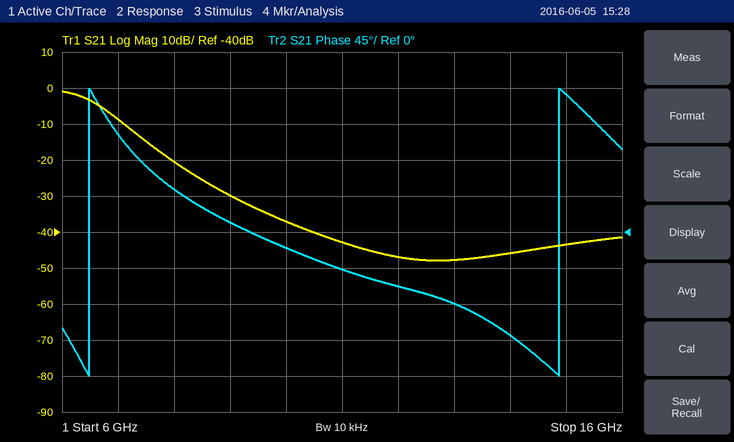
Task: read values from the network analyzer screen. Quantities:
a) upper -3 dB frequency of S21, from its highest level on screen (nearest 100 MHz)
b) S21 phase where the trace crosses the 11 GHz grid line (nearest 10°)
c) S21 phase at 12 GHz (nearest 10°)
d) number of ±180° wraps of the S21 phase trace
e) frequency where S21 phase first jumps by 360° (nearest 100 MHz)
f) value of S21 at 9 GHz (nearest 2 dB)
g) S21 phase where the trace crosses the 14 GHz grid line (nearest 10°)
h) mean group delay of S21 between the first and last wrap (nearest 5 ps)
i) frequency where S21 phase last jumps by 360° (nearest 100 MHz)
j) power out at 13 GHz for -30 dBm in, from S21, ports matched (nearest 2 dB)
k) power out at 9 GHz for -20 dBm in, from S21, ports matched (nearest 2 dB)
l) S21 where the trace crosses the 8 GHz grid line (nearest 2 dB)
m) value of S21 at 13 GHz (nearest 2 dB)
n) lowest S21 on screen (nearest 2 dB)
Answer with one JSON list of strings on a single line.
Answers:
["6.6 GHz", "-50°", "-70°", "2", "6.5 GHz", "-30 dB", "-130°", "120 ps", "14.9 GHz", "-78 dBm", "-50 dBm", "-20 dB", "-48 dB", "-48 dB"]
